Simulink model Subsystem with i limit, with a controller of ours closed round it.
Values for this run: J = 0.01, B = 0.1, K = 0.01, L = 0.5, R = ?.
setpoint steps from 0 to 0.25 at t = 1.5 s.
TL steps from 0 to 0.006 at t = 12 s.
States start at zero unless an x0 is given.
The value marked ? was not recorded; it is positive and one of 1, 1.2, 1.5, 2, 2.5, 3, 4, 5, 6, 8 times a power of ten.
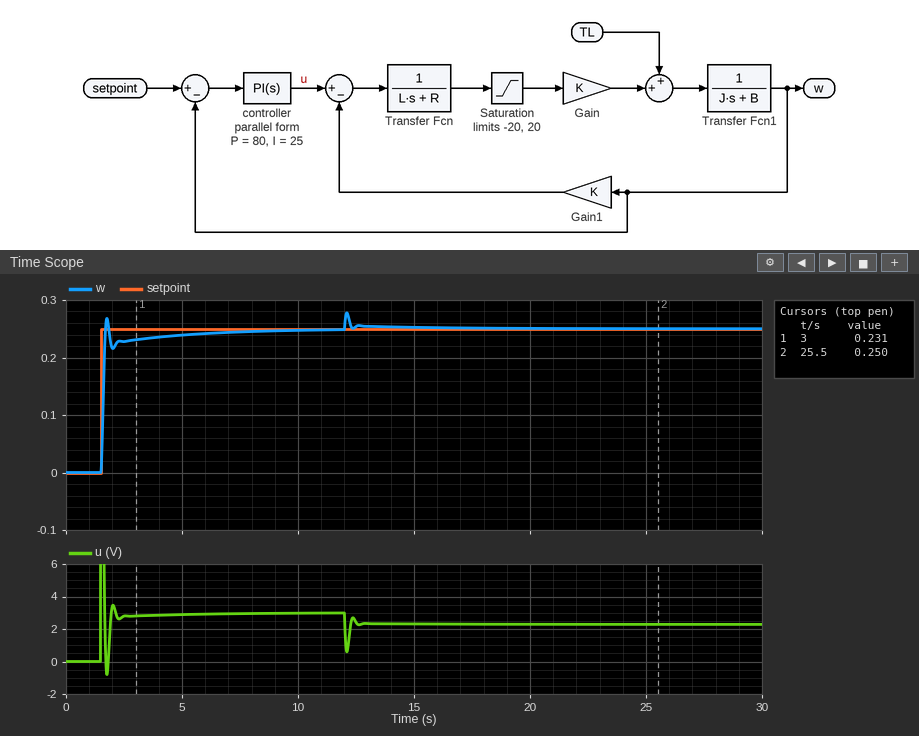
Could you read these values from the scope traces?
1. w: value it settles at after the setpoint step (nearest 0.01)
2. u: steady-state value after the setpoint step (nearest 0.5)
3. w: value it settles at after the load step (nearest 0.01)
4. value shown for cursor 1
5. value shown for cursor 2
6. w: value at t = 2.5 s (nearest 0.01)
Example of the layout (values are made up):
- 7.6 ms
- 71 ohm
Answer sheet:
- 0.25
- 3.0
- 0.25
- 0.231
- 0.250
- 0.23
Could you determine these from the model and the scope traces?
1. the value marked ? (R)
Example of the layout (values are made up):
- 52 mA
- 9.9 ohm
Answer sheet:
- 1.2
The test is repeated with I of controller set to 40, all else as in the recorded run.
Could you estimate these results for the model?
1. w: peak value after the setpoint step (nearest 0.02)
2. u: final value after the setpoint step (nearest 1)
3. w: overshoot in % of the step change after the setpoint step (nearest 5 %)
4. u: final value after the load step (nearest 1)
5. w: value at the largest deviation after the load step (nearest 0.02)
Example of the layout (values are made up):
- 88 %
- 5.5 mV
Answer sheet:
- 0.28
- 3
- 10 %
- 2
- 0.28
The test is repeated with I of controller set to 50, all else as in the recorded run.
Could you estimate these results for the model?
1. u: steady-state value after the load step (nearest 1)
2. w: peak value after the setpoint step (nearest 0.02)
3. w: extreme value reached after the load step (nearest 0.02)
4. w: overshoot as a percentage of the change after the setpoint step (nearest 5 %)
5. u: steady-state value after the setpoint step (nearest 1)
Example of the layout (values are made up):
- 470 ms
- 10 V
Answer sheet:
- 2
- 0.28
- 0.28
- 10 %
- 3
